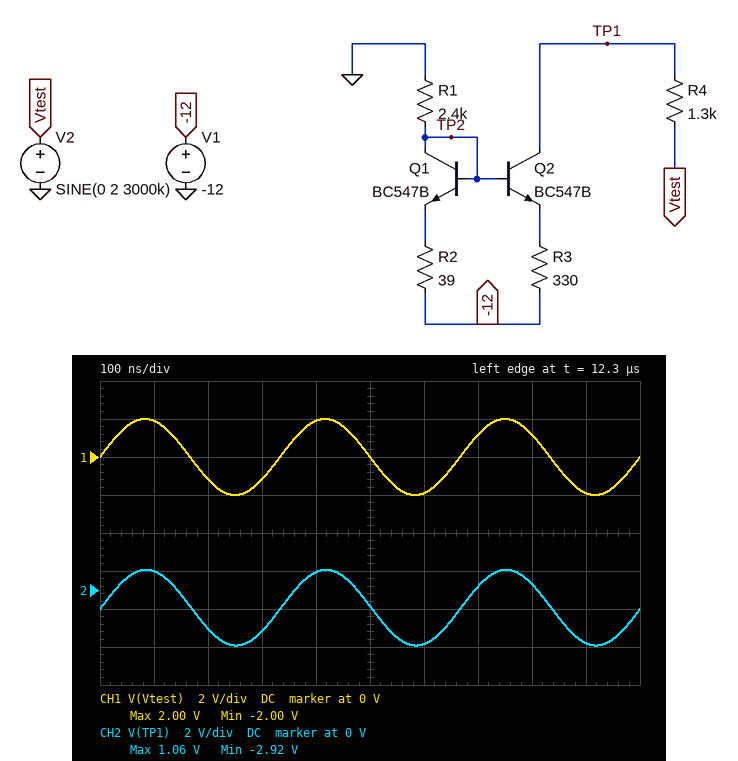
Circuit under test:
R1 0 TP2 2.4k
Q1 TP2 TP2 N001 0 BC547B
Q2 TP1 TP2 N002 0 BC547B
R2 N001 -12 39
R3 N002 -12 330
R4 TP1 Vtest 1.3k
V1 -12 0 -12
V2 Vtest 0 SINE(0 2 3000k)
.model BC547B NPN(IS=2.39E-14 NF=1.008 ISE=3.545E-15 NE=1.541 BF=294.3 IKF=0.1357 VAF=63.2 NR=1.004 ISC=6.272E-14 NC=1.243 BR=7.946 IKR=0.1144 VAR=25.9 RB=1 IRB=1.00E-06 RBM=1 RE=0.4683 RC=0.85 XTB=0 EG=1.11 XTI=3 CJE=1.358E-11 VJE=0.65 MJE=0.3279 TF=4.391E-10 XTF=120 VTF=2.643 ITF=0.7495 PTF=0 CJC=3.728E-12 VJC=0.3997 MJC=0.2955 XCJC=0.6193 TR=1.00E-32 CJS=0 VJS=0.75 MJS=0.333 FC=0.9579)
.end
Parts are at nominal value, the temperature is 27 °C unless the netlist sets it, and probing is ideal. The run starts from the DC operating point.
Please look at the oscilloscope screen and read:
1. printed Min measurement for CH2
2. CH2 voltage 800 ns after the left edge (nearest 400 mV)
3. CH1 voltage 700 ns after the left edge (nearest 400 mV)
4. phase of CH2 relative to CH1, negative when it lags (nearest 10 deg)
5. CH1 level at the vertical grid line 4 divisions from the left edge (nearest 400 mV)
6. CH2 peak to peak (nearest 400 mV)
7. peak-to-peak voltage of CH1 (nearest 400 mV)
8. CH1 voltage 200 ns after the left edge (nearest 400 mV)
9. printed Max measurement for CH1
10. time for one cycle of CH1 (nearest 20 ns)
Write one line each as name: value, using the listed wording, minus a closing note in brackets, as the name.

printed Min measurement for CH2: -2.92 V
CH2 voltage 800 ns after the left edge: 400 mV
CH1 voltage 700 ns after the left edge: 1.2 V
phase of CH2 relative to CH1, negative when it lags: 0 deg
CH1 level at the vertical grid line 4 divisions from the left edge: 2.0 V
CH2 peak to peak: 4.0 V
peak-to-peak voltage of CH1: 4.0 V
CH1 voltage 200 ns after the left edge: -1.2 V
printed Max measurement for CH1: 2.00 V
time for one cycle of CH1: 340 ns
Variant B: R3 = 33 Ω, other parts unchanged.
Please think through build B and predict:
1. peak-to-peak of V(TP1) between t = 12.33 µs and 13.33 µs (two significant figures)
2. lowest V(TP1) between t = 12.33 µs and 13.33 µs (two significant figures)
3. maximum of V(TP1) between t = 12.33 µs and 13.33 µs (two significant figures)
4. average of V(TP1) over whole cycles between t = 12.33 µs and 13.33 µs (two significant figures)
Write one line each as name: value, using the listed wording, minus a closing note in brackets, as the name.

peak-to-peak of V(TP1) between t = 12.33 µs and 13.33 µs: 3.9 V
lowest V(TP1) between t = 12.33 µs and 13.33 µs: -8.9 V
maximum of V(TP1) between t = 12.33 µs and 13.33 µs: -5.0 V
average of V(TP1) over whole cycles between t = 12.33 µs and 13.33 µs: -7.0 V
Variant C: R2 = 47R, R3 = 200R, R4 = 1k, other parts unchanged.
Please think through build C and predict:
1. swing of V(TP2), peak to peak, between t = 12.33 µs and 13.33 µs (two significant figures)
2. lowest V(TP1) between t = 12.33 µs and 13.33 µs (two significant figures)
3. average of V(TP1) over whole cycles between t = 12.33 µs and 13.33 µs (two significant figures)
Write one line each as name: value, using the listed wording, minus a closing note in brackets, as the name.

swing of V(TP2), peak to peak, between t = 12.33 µs and 13.33 µs: 5.7 mV
lowest V(TP1) between t = 12.33 µs and 13.33 µs: -3.3 V
average of V(TP1) over whole cycles between t = 12.33 µs and 13.33 µs: -1.3 V
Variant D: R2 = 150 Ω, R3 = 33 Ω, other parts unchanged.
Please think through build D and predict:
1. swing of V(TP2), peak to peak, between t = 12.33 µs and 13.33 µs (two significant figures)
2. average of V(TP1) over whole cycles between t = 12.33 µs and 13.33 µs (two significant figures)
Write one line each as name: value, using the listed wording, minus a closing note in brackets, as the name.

swing of V(TP2), peak to peak, between t = 12.33 µs and 13.33 µs: 81 mV
average of V(TP1) over whole cycles between t = 12.33 µs and 13.33 µs: -12 V
